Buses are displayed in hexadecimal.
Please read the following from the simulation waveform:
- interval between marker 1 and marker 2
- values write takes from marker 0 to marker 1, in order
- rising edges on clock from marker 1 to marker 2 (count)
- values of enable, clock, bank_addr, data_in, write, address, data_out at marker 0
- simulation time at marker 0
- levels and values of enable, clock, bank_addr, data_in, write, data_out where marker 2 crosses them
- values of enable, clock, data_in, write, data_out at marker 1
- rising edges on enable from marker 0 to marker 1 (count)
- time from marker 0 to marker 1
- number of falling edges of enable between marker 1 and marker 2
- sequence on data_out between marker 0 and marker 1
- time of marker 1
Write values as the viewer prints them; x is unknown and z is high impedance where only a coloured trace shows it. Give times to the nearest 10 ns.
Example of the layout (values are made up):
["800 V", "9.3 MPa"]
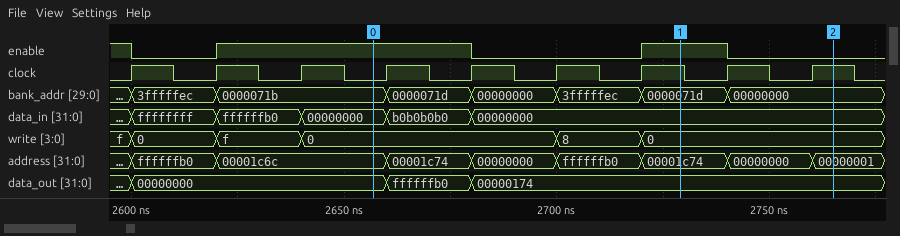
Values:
["40 ns", "0, 8, 0", "2", "enable=1, clock=0, bank_addr=0000071b, data_in=00000000, write=0, address=00001c6c, data_out=00000000", "2660 ns", "enable=0, clock=1, bank_addr=00000000, data_in=00000000, write=0, data_out=00000174", "enable=1, clock=1, data_in=00000000, write=0, data_out=00000174", "1", "70 ns", "1", "00000000, ffffffb0, 00000174", "2730 ns"]
